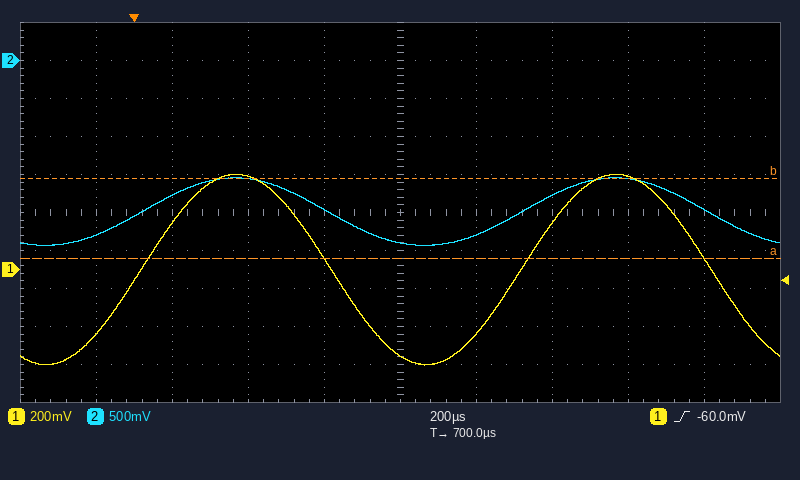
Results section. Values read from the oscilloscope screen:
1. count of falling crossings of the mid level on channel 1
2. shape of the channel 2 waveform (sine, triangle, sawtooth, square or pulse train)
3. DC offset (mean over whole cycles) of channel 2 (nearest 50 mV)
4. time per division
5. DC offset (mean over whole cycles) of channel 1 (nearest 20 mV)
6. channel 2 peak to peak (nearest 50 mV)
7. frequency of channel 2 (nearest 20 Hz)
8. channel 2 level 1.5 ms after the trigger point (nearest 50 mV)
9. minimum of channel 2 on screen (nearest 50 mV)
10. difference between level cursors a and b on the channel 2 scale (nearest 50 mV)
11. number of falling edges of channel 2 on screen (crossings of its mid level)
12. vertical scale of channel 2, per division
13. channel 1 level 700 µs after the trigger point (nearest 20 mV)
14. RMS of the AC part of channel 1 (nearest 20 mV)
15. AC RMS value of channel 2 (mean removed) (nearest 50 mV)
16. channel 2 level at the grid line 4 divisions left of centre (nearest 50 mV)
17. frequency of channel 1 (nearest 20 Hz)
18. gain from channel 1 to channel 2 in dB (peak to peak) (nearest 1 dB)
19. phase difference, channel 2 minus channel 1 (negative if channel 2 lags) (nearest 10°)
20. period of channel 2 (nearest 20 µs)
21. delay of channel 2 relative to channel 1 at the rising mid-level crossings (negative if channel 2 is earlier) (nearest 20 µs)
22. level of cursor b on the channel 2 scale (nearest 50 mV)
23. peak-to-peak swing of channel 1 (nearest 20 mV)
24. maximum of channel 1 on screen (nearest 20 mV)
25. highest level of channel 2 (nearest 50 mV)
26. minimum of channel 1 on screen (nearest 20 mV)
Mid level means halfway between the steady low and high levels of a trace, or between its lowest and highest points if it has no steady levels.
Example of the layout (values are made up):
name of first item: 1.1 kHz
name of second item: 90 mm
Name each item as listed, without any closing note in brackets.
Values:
count of falling crossings of the mid level on channel 1: 2
shape of the channel 2 waveform: sine
DC offset (mean over whole cycles) of channel 2: -2.00 V
time per division: 200 µs
DC offset (mean over whole cycles) of channel 1: 0 mV
channel 2 peak to peak: 900 mV
frequency of channel 2: 1.00 kHz
channel 2 level 1.5 ms after the trigger point: -1.95 V
minimum of channel 2 on screen: -2.45 V
difference between level cursors a and b on the channel 2 scale: 1.05 V
number of falling edges of channel 2 on screen: 2
vertical scale of channel 2, per division: 500 mV
channel 1 level 700 µs after the trigger point: -460 mV
RMS of the AC part of channel 1: 360 mV
AC RMS value of channel 2 (mean removed): 300 mV
channel 2 level at the grid line 4 divisions left of centre: -2.30 V
frequency of channel 1: 1.00 kHz
gain from channel 1 to channel 2 in dB (peak to peak): -1 dB
phase difference, channel 2 minus channel 1 (negative if channel 2 lags): 0°
period of channel 2: 1.00 ms
delay of channel 2 relative to channel 1 at the rising mid-level crossings (negative if channel 2 is earlier): 0 µs
level of cursor b on the channel 2 scale: -1.55 V
peak-to-peak swing of channel 1: 1.00 V
maximum of channel 1 on screen: 500 mV
highest level of channel 2: -1.55 V
minimum of channel 1 on screen: -500 mV
